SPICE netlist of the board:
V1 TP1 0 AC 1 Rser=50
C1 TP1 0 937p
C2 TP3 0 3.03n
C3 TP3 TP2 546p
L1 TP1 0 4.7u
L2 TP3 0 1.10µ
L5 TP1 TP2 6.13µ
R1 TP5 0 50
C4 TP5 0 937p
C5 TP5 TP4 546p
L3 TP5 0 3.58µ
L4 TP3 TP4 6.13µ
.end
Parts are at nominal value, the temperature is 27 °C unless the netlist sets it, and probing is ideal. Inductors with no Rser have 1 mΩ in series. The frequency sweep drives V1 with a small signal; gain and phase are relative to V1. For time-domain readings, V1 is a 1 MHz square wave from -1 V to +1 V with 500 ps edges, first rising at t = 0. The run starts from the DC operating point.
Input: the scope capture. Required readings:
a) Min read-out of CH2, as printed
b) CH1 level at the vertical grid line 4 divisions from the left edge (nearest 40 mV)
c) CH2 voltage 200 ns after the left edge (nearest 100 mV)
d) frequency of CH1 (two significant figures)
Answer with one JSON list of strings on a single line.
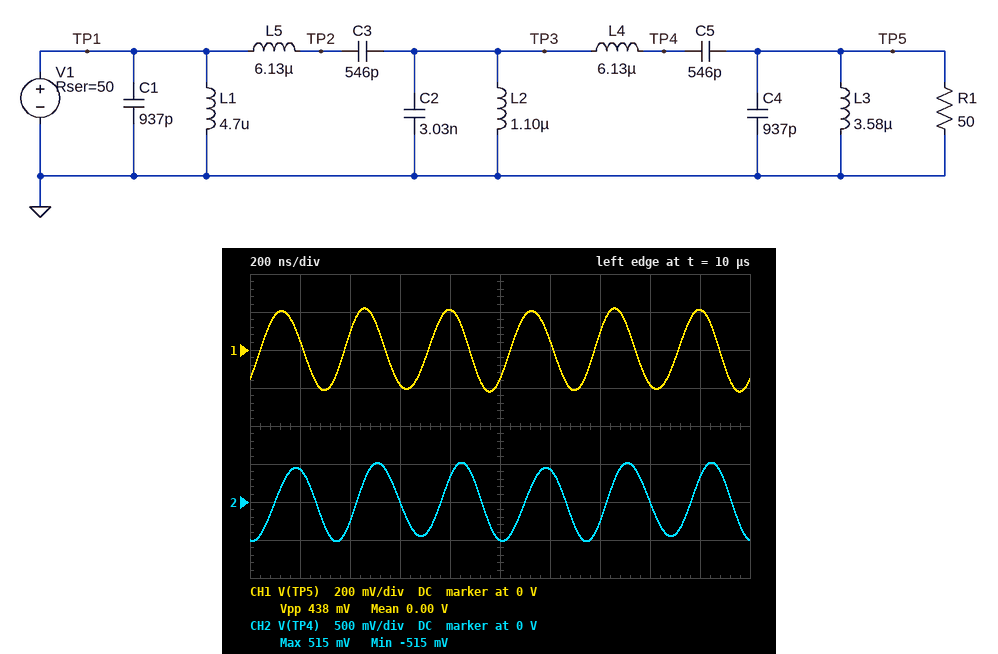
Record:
["-515 mV", "200 mV", "400 mV", "3.0 MHz"]
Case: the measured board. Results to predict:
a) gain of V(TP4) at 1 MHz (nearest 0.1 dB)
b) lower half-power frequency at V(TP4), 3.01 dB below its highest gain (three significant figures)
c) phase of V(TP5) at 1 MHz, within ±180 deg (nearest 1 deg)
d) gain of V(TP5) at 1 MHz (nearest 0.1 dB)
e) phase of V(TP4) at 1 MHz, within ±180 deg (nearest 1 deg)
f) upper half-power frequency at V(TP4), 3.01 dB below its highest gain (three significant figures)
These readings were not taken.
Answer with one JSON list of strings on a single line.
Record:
["-32.0 dB", "1.87 MHz", "20 deg", "-53.4 dB", "-130 deg", "3.95 MHz"]
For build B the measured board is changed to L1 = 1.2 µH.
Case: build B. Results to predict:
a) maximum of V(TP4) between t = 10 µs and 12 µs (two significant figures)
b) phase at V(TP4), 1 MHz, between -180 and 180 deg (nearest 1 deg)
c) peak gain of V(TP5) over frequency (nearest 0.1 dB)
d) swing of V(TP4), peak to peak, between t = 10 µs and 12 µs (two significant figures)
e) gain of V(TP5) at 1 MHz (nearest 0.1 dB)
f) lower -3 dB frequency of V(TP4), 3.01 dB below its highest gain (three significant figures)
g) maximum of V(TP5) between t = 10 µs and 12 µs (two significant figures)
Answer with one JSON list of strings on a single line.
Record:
["420 mV", "-100 deg", "-7.5 dB", "840 mV", "-65.4 dB", "1.93 MHz", "180 mV"]
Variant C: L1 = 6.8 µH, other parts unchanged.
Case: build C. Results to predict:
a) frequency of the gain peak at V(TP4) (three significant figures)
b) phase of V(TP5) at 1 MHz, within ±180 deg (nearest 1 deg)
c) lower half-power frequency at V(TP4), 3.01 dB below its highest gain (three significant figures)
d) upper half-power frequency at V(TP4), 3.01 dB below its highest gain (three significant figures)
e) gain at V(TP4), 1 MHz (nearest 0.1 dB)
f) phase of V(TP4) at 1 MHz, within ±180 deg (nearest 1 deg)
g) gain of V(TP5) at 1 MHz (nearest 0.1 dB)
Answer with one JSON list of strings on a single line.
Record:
["2.14 MHz", "4 deg", "1.89 MHz", "3.98 MHz", "-29.7 dB", "-147 deg", "-51.2 dB"]
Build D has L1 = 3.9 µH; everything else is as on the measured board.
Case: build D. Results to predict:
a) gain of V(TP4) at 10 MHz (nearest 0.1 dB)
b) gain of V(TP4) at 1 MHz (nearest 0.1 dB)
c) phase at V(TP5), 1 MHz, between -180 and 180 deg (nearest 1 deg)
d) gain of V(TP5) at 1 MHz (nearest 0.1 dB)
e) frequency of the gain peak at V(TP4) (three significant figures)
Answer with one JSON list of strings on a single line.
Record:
["-62.0 dB", "-33.4 dB", "27 deg", "-54.8 dB", "2.08 MHz"]
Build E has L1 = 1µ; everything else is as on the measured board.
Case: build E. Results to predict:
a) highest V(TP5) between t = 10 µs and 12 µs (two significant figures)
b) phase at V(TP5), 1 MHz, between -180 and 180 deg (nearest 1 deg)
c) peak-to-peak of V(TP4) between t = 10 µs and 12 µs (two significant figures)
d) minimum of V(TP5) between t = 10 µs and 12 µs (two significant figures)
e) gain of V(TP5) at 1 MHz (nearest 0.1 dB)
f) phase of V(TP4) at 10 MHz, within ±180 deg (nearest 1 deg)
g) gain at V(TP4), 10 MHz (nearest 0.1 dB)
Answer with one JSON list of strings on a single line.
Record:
["160 mV", "52 deg", "750 mV", "-160 mV", "-67.1 dB", "-55 deg", "-60.1 dB"]
